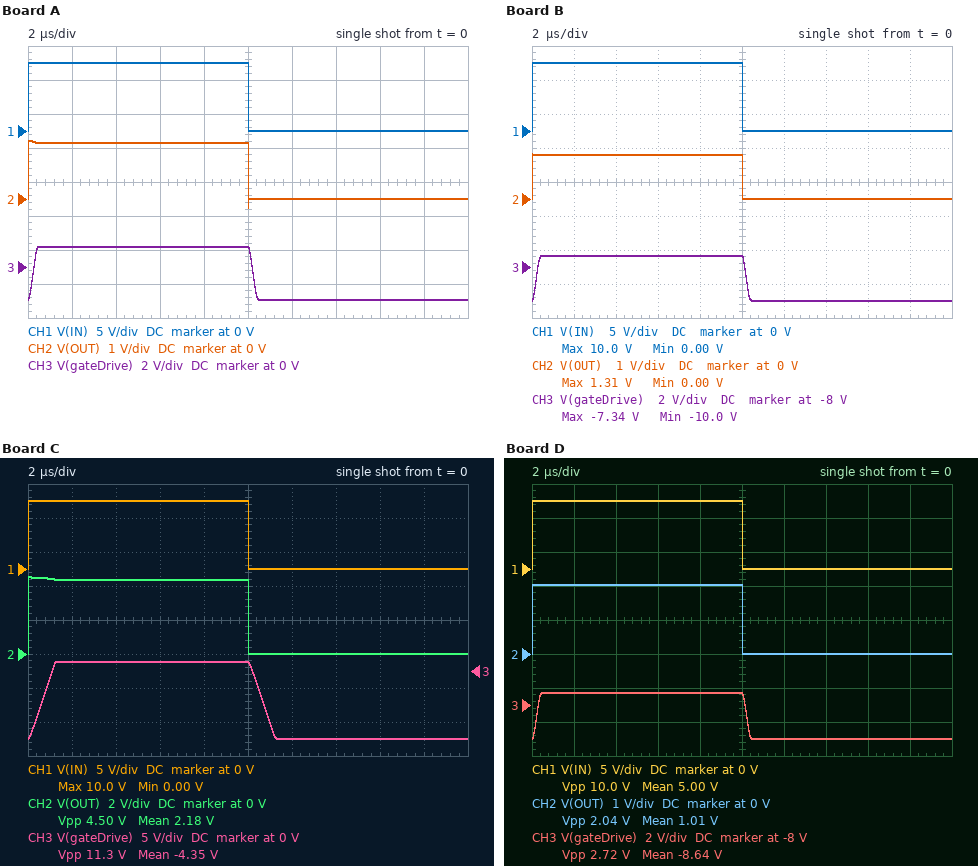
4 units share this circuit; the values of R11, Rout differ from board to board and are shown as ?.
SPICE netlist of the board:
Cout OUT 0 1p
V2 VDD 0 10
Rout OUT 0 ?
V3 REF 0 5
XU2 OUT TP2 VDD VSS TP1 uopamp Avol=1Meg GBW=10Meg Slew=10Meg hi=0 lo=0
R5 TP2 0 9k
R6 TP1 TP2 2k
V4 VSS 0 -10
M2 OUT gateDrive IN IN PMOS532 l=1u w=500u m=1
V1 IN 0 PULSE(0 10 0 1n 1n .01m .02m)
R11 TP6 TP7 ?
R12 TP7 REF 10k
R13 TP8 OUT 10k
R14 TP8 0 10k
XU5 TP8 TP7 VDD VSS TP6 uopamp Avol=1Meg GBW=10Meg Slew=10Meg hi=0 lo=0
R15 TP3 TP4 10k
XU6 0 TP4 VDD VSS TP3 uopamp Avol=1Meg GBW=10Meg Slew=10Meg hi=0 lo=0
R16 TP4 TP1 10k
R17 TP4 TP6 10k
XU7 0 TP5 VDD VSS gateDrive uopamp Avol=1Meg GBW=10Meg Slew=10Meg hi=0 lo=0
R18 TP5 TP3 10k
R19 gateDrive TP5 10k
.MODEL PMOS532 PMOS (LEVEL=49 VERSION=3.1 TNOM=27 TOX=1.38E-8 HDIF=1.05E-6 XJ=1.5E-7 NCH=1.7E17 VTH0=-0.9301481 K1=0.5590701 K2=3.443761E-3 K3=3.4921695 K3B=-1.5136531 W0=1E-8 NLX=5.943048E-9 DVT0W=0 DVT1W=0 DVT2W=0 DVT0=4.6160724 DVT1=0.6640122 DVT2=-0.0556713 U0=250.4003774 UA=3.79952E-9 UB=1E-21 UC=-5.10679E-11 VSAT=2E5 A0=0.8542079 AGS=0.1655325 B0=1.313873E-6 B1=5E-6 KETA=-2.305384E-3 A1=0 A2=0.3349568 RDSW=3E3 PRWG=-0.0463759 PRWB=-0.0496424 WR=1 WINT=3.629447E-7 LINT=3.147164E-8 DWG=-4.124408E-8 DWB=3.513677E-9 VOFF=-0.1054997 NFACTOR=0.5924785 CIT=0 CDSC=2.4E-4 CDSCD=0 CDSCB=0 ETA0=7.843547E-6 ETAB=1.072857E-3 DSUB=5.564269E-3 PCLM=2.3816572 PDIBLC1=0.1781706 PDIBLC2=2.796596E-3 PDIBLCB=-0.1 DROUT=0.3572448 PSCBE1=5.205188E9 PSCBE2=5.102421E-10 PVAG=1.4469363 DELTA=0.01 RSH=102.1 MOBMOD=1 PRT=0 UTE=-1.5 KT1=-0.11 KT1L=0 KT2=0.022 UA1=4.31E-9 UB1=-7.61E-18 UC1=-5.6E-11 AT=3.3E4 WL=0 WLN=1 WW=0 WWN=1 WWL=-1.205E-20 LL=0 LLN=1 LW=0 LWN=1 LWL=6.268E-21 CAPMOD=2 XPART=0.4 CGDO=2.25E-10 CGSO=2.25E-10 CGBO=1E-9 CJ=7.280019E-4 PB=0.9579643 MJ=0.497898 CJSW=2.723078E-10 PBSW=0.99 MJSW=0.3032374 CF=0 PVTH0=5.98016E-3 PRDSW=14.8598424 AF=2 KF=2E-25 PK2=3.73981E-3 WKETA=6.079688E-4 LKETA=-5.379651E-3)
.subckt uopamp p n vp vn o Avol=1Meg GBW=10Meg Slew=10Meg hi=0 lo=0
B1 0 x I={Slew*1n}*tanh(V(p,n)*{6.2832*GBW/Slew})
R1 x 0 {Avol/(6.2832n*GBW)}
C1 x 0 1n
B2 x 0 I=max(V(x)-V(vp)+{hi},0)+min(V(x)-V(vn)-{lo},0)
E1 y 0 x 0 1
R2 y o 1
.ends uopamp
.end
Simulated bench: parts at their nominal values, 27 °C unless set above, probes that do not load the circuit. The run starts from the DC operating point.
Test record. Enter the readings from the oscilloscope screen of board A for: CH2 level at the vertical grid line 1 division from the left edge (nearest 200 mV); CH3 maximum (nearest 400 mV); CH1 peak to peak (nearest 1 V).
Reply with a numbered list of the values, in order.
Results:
1. 1.6 V
2. 1.2 V
3. 10 V
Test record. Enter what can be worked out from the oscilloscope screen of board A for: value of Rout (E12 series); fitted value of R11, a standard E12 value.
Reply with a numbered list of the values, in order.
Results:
1. 47 Ω
2. 3.9 kΩ
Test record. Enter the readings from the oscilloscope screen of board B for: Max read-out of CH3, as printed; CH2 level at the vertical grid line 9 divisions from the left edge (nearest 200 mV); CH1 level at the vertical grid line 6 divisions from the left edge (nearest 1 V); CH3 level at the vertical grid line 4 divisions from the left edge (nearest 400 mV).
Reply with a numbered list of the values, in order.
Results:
1. -7.34 V
2. 0 V
3. 0 V
4. -7.2 V
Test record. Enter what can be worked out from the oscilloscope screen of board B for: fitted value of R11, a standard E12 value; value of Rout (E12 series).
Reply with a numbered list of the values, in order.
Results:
1. 22 kΩ
2. 33 Ω
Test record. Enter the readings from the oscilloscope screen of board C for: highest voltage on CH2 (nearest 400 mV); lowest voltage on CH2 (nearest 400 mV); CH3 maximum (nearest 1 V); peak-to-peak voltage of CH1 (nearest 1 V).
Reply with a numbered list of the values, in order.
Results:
1. 4.4 V
2. 0 V
3. 1 V
4. 10 V
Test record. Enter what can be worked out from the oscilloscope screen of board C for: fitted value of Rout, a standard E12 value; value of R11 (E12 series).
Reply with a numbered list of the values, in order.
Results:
1. 180 Ω
2. 22 kΩ
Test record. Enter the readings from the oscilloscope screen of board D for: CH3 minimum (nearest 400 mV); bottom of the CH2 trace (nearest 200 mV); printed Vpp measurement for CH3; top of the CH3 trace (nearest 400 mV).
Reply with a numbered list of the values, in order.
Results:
1. -10.0 V
2. 0 V
3. 2.72 V
4. -7.2 V
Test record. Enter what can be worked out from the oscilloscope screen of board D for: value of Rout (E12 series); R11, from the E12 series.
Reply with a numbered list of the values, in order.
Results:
1. 56 Ω
2. 27 kΩ
